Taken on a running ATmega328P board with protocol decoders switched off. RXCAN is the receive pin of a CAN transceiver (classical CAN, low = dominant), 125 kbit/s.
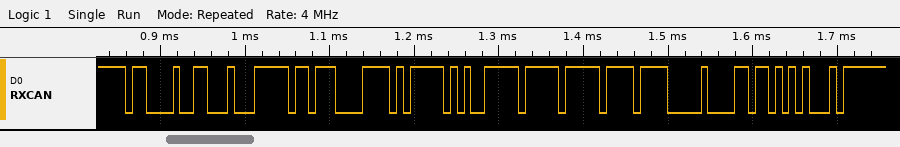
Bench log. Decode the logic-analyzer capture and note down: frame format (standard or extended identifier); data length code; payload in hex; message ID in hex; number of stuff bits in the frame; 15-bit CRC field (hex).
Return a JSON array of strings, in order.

["standard", "8", "FE E1 EB F4 FF FF EF 00", "0x613", "6", "0x36A8"]
